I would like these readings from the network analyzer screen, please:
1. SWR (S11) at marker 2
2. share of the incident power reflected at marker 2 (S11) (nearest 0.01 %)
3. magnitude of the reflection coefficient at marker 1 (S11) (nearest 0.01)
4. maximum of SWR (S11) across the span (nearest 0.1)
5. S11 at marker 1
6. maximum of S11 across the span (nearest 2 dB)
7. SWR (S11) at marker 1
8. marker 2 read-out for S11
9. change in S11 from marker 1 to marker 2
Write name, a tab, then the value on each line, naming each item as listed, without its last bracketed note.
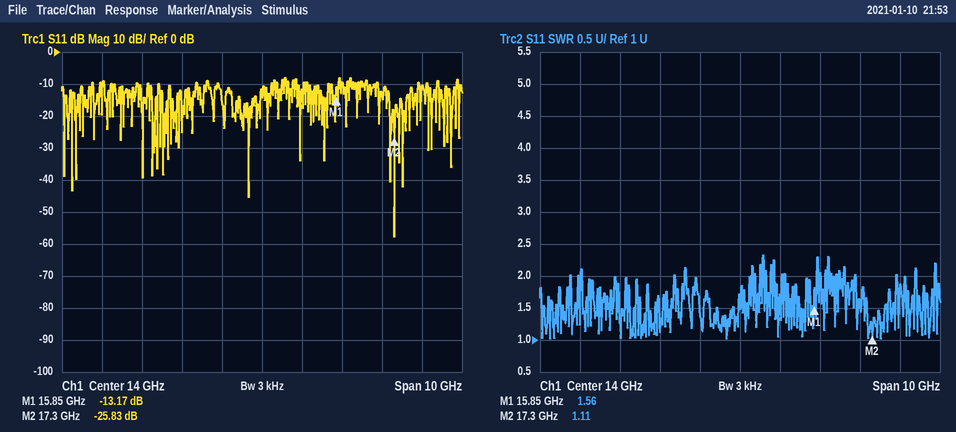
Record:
SWR (S11) at marker 2	1.11
share of the incident power reflected at marker 2 (S11)	0.26 %
magnitude of the reflection coefficient at marker 1 (S11)	0.22
maximum of SWR (S11) across the span	2.3
S11 at marker 1	-13.17 dB
maximum of S11 across the span	-8 dB
SWR (S11) at marker 1	1.56
marker 2 read-out for S11	-25.83 dB
change in S11 from marker 1 to marker 2	-12.66 dB
